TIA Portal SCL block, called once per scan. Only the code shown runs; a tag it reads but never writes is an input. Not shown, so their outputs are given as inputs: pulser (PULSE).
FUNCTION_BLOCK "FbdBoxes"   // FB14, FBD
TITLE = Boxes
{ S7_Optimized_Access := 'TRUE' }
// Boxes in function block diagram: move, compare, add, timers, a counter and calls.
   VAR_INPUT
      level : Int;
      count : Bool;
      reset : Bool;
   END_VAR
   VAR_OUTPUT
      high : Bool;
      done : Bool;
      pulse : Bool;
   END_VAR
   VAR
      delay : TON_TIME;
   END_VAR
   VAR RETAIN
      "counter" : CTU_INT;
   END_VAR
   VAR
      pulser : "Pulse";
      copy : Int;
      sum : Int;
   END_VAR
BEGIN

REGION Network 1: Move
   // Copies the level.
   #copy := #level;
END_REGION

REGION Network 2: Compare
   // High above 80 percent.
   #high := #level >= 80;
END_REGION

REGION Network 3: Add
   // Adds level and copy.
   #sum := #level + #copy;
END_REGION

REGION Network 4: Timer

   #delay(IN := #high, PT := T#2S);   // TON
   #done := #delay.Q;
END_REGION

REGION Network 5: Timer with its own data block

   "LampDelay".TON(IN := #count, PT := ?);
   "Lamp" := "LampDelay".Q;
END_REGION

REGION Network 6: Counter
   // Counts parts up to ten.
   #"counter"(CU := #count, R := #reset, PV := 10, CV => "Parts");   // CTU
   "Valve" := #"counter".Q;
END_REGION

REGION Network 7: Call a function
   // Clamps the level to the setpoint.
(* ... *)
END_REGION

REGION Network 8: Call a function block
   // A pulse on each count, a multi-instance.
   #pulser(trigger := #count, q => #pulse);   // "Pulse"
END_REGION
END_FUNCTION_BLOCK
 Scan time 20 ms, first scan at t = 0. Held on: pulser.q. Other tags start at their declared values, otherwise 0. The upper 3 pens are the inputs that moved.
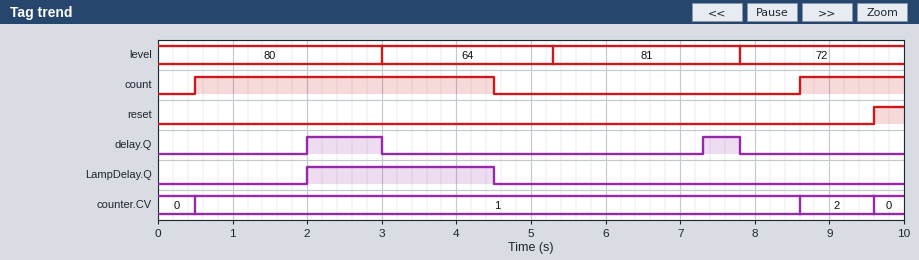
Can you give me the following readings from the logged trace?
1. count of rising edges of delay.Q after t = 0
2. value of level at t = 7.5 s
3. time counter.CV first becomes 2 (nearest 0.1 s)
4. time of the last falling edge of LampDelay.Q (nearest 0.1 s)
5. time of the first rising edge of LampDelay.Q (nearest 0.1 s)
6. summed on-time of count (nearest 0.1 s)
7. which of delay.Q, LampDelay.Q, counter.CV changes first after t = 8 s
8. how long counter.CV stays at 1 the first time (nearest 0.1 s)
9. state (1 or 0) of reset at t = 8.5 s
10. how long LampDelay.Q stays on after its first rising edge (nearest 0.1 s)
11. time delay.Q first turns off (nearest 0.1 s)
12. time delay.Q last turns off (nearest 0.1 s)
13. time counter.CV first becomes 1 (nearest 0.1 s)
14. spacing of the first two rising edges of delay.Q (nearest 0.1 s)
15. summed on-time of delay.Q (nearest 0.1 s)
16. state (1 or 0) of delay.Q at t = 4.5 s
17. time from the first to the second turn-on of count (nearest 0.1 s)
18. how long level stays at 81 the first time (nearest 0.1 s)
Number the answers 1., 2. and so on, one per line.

1. 2
2. 81
3. 8.6 s
4. 4.5 s
5. 2.0 s
6. 5.4 s
7. counter.CV
8. 8.1 s
9. 0
10. 2.5 s
11. 3.0 s
12. 7.8 s
13. 0.5 s
14. 5.3 s
15. 1.5 s
16. 0
17. 8.1 s
18. 2.5 s
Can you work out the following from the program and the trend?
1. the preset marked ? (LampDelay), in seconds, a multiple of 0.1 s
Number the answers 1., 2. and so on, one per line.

1. 1.5 s
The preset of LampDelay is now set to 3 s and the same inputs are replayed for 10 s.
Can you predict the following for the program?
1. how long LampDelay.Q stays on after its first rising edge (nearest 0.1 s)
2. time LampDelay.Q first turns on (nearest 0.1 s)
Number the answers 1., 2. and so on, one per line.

1. 1.0 s
2. 3.5 s
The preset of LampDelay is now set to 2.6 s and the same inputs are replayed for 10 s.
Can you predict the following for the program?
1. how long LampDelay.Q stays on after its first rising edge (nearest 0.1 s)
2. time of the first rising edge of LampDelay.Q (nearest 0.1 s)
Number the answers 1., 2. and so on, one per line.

1. 1.4 s
2. 3.1 s
